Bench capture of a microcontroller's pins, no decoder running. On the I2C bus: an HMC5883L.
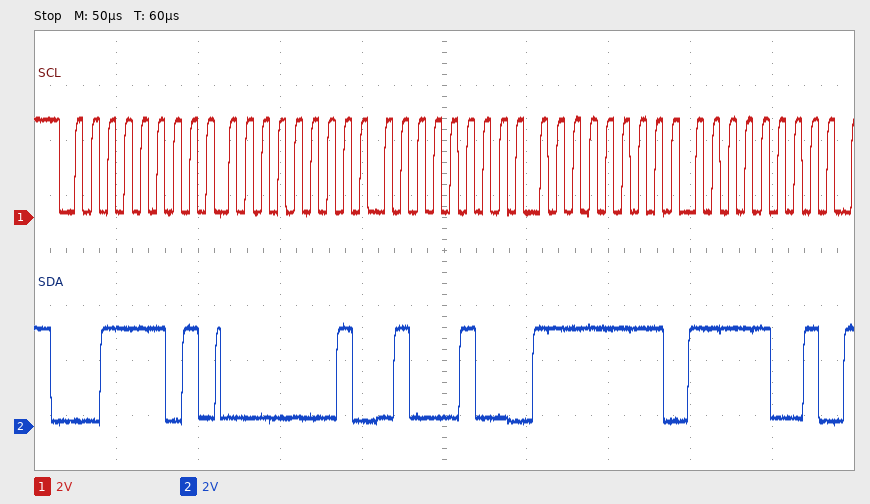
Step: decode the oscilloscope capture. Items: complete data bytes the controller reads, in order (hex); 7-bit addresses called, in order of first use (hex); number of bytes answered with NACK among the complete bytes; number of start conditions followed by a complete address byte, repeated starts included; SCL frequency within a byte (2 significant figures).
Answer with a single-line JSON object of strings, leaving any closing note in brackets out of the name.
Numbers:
{"complete data bytes the controller reads, in order": "01 44 FF F9", "7-bit addresses called, in order of first use": "0x1E", "number of bytes answered with NACK among the complete bytes": "0", "number of start conditions followed by a complete address byte, repeated starts included": "1", "SCL frequency within a byte": "100 kHz"}
